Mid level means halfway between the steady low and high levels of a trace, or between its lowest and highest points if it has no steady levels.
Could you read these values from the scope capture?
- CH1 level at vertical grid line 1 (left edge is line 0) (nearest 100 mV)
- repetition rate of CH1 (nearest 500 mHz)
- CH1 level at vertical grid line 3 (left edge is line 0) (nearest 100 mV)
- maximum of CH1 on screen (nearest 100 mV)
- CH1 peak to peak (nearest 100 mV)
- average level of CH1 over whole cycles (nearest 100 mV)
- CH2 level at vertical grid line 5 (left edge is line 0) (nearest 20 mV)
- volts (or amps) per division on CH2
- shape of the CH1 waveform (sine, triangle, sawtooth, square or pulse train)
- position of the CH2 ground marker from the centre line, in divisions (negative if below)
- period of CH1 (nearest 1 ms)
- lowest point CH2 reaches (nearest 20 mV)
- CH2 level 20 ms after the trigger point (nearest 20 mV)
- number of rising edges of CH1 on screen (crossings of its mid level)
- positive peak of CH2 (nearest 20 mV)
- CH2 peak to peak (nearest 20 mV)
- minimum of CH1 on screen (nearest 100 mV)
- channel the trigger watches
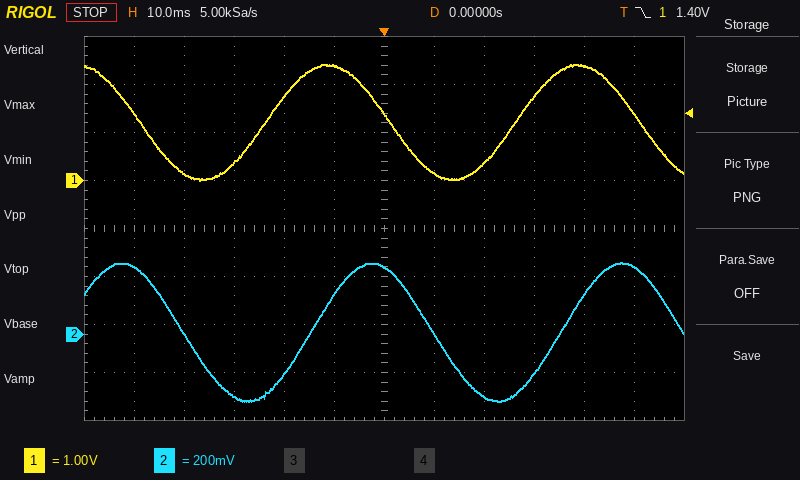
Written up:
1.4 V
20.0 Hz
400 mV
2.4 V
2.4 V
1.2 V
160 mV
200 mV
sine
-2.2 div
50 ms
-280 mV
-260 mV
2
300 mV
580 mV
0.0 V
CH1
